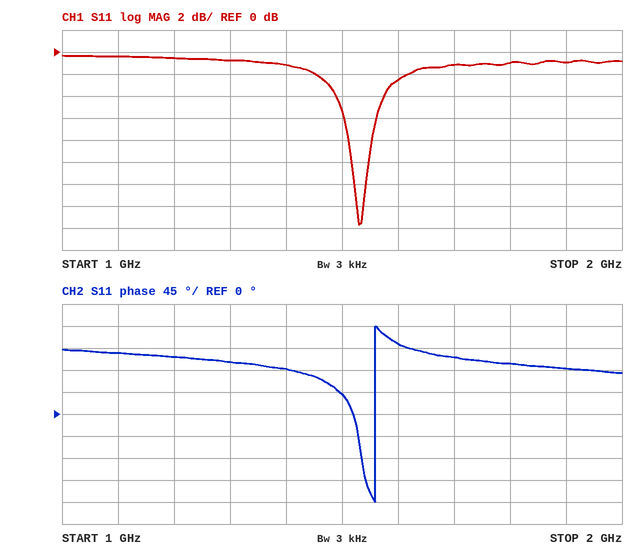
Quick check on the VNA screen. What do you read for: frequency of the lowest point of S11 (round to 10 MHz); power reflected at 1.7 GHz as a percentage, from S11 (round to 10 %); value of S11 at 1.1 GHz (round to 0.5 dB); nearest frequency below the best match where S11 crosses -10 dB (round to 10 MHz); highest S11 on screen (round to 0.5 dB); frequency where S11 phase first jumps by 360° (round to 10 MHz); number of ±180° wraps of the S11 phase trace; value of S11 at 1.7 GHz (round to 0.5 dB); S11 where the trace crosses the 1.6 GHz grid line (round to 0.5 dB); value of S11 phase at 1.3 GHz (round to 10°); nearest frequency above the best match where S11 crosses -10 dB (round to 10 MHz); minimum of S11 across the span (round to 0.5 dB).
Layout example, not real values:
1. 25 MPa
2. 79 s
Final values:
1. 1.53 GHz
2. 80 %
3. -0.5 dB
4. 1.52 GHz
5. -0.5 dB
6. 1.56 GHz
7. 1
8. -1.0 dB
9. -2.5 dB
10. 110°
11. 1.55 GHz
12. -15.5 dB
